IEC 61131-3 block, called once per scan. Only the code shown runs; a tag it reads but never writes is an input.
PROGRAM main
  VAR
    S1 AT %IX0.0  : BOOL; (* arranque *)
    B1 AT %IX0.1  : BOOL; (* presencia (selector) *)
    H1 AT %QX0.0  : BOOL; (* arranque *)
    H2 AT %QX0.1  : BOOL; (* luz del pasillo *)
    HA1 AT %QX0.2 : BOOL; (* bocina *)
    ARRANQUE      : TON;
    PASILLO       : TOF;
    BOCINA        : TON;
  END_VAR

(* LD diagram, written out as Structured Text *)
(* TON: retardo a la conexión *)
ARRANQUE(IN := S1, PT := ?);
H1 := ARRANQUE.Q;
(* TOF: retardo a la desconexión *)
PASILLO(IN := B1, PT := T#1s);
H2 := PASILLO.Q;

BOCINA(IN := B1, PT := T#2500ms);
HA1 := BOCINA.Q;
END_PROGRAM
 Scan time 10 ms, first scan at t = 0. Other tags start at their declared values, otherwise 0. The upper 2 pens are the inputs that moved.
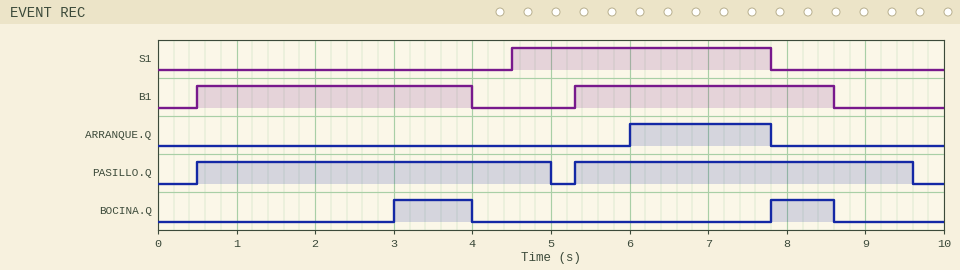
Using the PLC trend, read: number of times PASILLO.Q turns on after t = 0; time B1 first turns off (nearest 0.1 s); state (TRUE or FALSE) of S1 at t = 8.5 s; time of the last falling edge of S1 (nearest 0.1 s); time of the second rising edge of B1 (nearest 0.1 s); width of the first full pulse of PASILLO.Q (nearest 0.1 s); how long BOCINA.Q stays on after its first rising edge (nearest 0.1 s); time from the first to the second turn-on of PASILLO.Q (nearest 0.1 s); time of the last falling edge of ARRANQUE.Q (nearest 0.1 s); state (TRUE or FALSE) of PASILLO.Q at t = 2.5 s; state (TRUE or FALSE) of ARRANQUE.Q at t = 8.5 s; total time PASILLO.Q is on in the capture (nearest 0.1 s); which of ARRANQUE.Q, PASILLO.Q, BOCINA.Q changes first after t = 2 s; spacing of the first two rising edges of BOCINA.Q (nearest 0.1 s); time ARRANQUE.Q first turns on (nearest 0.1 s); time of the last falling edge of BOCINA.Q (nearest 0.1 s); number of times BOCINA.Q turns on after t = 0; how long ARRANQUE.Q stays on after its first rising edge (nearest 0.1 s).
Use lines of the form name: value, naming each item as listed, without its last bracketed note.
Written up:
number of times PASILLO.Q turns on after t = 0: 2
time B1 first turns off: 4.0 s
state (TRUE or FALSE) of S1 at t = 8.5 s: FALSE
time of the last falling edge of S1: 7.8 s
time of the second rising edge of B1: 5.3 s
width of the first full pulse of PASILLO.Q: 4.5 s
how long BOCINA.Q stays on after its first rising edge: 1.0 s
time from the first to the second turn-on of PASILLO.Q: 4.8 s
time of the last falling edge of ARRANQUE.Q: 7.8 s
state (TRUE or FALSE) of PASILLO.Q at t = 2.5 s: TRUE
state (TRUE or FALSE) of ARRANQUE.Q at t = 8.5 s: FALSE
total time PASILLO.Q is on in the capture: 8.8 s
which of ARRANQUE.Q, PASILLO.Q, BOCINA.Q changes first after t = 2 s: BOCINA.Q
spacing of the first two rising edges of BOCINA.Q: 4.8 s
time ARRANQUE.Q first turns on: 6.0 s
time of the last falling edge of BOCINA.Q: 8.6 s
number of times BOCINA.Q turns on after t = 0: 2
how long ARRANQUE.Q stays on after its first rising edge: 1.8 s
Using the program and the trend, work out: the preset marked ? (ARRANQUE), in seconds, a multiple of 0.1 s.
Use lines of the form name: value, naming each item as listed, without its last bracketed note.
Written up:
the preset marked ? (ARRANQUE), in seconds, a multiple of 0.1 s: 1.5 s
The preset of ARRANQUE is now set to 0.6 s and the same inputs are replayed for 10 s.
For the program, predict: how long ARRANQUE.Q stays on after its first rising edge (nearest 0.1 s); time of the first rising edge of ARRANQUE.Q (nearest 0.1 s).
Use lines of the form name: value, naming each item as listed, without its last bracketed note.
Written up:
how long ARRANQUE.Q stays on after its first rising edge: 2.7 s
time of the first rising edge of ARRANQUE.Q: 5.1 s
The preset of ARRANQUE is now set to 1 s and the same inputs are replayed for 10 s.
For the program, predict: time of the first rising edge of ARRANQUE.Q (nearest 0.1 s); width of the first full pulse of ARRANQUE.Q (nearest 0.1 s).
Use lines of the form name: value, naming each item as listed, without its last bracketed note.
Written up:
time of the first rising edge of ARRANQUE.Q: 5.5 s
width of the first full pulse of ARRANQUE.Q: 2.3 s
